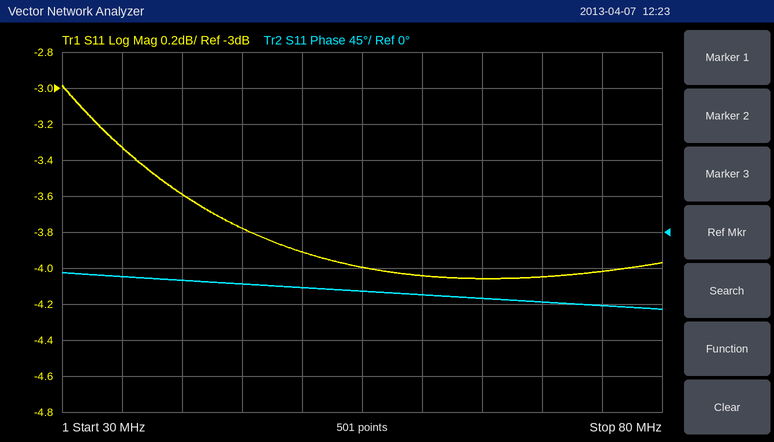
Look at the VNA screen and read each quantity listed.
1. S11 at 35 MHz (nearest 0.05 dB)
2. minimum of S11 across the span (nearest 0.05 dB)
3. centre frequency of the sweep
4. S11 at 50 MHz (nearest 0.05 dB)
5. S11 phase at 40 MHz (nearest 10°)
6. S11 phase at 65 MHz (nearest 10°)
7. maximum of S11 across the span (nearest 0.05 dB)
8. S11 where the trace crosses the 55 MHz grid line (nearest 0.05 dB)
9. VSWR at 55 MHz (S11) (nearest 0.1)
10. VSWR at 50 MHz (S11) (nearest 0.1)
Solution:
-3.35 dB
-4.05 dB
55 MHz
-3.90 dB
-60°
-80°
-3.00 dB
-4.00 dB
4.4
4.5
